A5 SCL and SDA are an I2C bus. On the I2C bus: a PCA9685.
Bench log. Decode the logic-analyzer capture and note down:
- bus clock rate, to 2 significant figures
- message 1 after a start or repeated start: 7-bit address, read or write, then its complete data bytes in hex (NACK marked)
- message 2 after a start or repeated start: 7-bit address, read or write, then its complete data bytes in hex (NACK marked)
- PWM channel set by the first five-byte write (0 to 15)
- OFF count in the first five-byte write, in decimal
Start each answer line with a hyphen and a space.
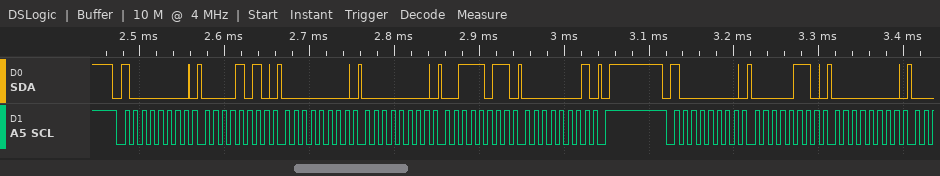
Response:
- 100 kHz
- 0x40 write: 0A 00 00 3B 01
- 0x40 write: 06 00
- 1
- 315
